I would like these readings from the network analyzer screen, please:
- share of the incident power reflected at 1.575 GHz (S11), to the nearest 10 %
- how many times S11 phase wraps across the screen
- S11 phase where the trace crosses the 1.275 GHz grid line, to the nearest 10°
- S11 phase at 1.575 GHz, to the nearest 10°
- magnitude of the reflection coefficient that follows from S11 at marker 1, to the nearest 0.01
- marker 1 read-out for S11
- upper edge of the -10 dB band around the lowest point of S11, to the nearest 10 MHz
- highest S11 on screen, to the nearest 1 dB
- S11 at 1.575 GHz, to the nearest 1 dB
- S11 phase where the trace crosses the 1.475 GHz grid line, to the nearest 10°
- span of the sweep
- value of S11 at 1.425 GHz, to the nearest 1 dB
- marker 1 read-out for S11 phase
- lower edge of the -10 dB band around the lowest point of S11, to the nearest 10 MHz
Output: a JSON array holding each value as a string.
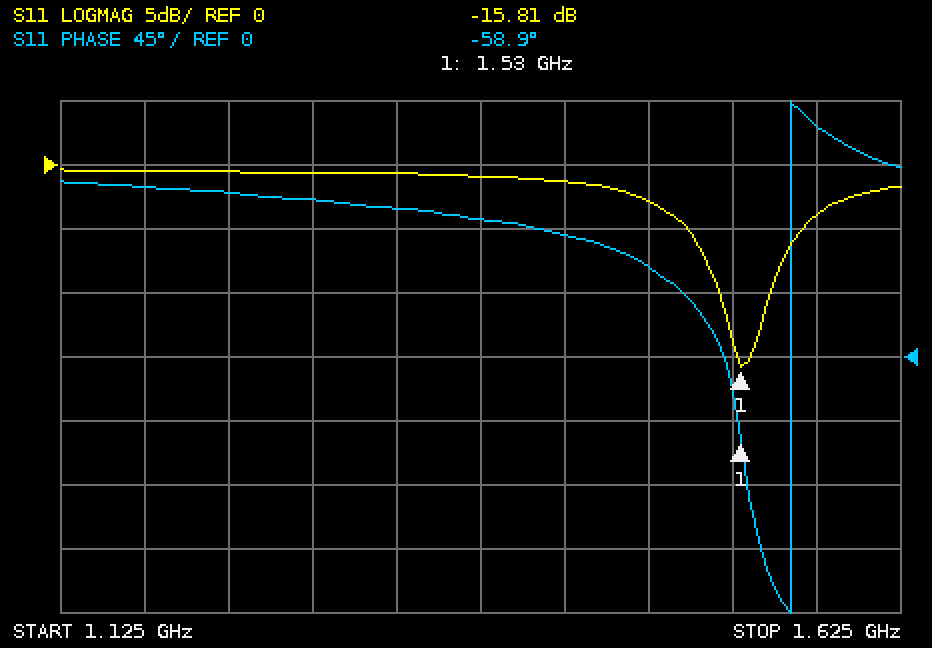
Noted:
["40 %", "1", "110°", "160°", "0.16", "-15.81 dB", "1.55 GHz", "0 dB", "-4 dB", "60°", "500 MHz", "-1 dB", "-58.9°", "1.52 GHz"]
